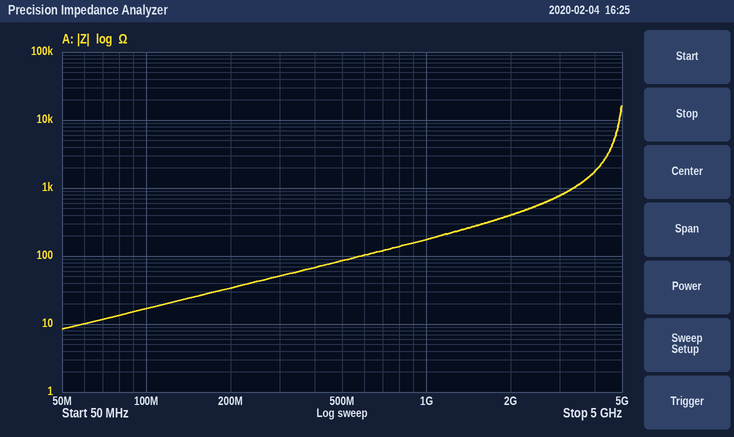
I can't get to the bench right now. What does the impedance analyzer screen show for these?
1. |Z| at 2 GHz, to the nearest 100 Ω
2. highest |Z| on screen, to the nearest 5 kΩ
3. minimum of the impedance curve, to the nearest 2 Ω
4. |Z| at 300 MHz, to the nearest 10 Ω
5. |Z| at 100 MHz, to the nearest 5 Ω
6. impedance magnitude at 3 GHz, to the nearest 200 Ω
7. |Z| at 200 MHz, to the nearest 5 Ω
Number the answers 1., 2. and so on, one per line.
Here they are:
1. 400 Ω
2. 15 kΩ
3. 8 Ω
4. 50 Ω
5. 15 Ω
6. 800 Ω
7. 35 Ω
